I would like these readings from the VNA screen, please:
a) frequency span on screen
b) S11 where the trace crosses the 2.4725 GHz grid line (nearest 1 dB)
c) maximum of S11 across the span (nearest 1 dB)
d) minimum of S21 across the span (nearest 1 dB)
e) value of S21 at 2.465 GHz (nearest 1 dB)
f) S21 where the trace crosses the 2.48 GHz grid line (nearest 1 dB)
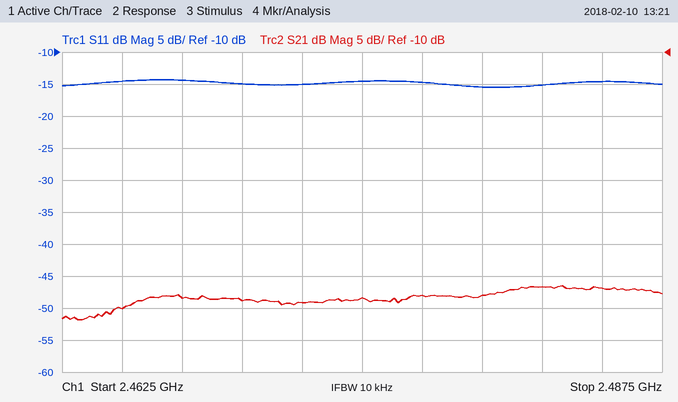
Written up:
25 MHz
-15 dB
-14 dB
-52 dB
-50 dB
-48 dB
